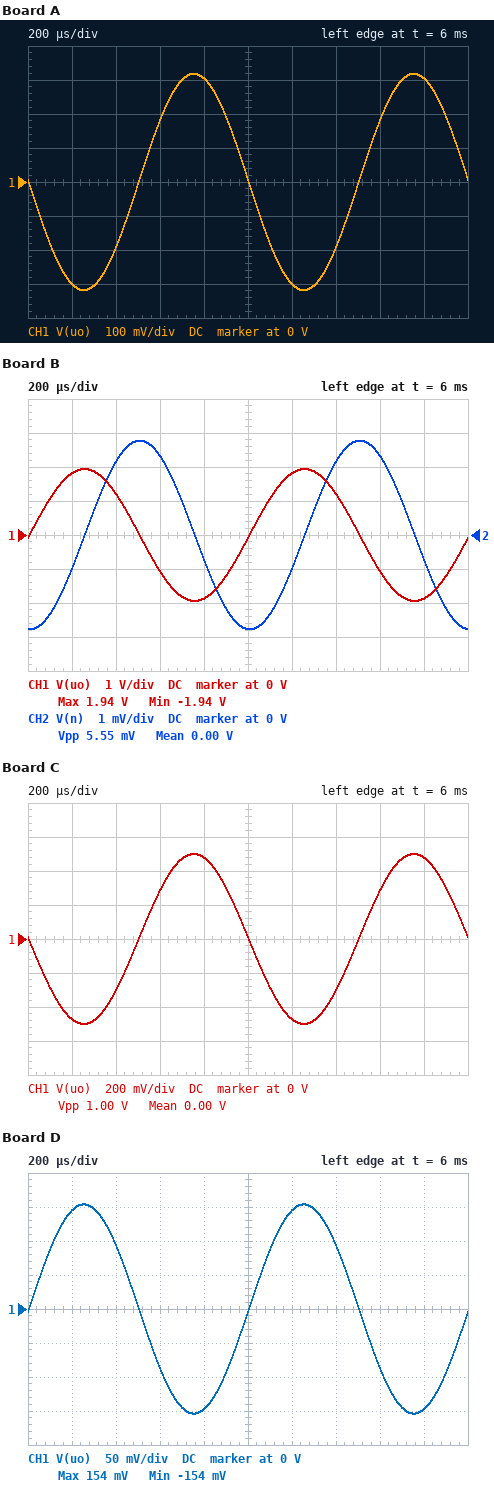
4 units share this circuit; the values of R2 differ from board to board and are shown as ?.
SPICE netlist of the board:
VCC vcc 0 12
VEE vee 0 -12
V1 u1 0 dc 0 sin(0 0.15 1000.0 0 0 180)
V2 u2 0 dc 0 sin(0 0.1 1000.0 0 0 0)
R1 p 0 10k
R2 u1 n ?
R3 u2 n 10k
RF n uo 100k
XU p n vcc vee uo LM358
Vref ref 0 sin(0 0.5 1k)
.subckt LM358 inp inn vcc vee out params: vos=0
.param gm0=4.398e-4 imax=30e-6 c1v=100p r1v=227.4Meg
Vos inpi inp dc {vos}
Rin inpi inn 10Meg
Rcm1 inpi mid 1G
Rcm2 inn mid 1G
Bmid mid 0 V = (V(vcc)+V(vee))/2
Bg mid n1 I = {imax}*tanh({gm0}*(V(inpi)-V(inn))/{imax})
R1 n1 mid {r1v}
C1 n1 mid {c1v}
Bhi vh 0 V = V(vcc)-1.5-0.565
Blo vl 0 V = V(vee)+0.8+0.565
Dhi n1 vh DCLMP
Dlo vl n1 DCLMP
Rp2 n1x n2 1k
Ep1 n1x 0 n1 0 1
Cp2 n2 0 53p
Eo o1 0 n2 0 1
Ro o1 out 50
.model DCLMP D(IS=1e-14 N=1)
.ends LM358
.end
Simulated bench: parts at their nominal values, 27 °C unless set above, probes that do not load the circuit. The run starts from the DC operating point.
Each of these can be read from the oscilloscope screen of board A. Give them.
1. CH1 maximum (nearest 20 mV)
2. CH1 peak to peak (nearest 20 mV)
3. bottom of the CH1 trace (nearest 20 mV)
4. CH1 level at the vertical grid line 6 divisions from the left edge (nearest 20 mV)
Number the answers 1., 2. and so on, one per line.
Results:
1. 320 mV
2. 640 mV
3. -320 mV
4. -300 mV
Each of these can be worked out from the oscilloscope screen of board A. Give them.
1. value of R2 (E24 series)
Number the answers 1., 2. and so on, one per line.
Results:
1. 22 kΩ
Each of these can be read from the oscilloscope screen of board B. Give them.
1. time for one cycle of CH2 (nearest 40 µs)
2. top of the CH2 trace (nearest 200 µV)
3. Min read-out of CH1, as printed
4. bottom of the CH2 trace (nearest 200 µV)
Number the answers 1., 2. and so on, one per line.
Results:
1. 1.00 ms
2. 2.8 mV
3. -1.94 V
4. -2.8 mV
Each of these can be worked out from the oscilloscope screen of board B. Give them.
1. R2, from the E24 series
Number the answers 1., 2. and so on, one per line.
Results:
1. 5.1 kΩ
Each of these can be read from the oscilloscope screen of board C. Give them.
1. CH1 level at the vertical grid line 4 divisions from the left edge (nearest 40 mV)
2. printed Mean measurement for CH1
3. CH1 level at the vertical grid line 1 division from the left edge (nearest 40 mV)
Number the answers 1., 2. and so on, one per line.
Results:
1. 480 mV
2. 0.00 V
3. -480 mV
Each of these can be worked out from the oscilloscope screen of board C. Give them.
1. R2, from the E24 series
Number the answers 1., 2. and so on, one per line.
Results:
1. 30 kΩ
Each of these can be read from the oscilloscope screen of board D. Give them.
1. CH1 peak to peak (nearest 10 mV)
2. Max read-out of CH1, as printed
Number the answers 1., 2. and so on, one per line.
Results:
1. 310 mV
2. 154 mV
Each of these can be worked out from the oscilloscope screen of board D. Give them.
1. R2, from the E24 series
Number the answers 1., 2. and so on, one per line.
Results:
1. 13 kΩ
